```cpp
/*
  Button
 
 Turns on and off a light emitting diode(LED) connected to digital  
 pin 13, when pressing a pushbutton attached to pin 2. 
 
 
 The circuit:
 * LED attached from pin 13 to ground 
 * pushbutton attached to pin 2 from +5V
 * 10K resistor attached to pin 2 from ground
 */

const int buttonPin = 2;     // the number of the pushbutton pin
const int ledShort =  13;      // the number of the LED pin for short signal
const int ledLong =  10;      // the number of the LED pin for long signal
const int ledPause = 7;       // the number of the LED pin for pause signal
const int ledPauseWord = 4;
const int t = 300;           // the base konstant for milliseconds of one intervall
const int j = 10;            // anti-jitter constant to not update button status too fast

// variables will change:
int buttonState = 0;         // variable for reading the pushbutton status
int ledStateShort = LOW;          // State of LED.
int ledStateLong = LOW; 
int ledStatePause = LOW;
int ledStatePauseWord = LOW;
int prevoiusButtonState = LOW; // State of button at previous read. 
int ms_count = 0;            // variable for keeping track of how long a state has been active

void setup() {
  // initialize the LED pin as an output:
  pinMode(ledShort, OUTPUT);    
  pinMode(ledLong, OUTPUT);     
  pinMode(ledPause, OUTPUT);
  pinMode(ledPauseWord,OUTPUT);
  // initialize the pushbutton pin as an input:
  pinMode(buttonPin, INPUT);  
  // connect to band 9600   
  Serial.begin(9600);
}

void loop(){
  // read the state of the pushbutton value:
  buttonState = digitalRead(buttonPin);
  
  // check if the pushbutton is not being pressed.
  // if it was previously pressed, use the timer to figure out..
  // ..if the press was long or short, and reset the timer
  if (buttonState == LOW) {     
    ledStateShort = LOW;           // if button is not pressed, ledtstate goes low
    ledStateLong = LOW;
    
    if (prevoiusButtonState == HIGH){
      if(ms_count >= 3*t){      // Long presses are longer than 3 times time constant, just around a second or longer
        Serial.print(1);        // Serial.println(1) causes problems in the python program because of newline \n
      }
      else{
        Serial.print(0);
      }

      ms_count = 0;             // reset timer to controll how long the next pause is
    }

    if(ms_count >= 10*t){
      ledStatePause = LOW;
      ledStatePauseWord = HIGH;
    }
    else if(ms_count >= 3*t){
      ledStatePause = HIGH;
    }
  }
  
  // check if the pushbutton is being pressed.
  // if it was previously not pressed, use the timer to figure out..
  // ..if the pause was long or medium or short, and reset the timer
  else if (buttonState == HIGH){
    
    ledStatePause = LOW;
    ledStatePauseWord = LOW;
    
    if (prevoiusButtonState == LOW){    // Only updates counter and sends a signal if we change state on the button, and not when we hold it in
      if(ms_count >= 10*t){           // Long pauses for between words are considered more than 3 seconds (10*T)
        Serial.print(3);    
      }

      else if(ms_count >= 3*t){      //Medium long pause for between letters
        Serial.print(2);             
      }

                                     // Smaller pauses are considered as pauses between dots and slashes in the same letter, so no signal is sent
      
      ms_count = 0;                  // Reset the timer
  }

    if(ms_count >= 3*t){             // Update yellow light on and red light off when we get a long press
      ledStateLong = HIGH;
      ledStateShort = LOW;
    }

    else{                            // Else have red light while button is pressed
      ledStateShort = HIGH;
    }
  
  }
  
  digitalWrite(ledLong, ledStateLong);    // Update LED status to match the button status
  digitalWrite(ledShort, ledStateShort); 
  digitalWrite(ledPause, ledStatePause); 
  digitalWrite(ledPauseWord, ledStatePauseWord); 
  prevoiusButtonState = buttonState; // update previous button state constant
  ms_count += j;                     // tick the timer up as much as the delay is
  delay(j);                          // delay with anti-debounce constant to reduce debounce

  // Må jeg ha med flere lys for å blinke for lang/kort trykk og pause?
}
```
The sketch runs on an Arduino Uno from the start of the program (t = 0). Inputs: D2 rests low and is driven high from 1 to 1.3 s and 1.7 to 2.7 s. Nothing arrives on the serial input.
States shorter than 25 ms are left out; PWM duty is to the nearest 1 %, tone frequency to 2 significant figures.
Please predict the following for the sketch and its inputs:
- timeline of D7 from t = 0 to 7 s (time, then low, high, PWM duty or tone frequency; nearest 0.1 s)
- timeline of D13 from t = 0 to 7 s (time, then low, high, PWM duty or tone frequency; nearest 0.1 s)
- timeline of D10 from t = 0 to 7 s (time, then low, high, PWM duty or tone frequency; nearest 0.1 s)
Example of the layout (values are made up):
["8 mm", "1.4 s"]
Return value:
["0 s low; 0.9 s high; 1 s low; 3.6 s high; 5.7 s low", "0 s low; 1 s high; 1.3 s low; 1.7 s high; 2.6 s low", "0 s low; 2.6 s high; 2.7 s low"]
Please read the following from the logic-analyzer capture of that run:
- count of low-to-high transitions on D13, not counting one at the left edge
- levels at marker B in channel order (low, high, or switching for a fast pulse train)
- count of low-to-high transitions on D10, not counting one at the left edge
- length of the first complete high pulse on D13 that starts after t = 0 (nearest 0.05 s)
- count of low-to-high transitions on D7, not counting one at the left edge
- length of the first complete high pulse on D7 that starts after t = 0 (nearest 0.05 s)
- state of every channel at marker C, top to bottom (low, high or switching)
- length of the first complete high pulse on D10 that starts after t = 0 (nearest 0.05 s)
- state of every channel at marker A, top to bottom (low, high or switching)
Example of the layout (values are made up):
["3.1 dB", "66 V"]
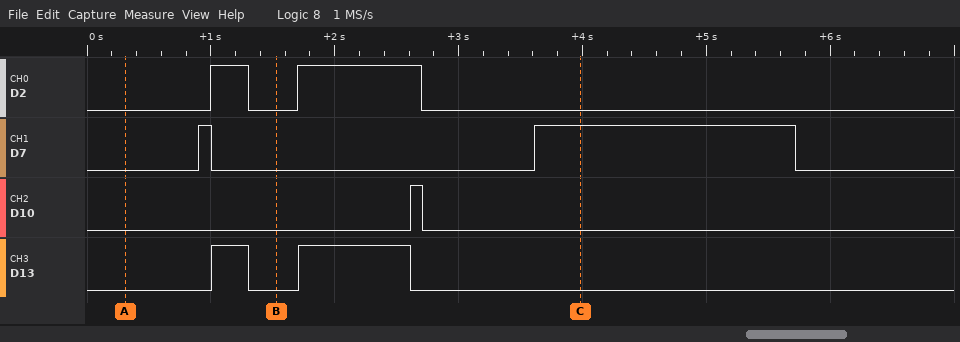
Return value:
["2", "D2 low, D7 low, D10 low, D13 low", "1", "0.30 s", "2", "0.10 s", "D2 low, D7 high, D10 low, D13 low", "0.10 s", "D2 low, D7 low, D10 low, D13 low"]
